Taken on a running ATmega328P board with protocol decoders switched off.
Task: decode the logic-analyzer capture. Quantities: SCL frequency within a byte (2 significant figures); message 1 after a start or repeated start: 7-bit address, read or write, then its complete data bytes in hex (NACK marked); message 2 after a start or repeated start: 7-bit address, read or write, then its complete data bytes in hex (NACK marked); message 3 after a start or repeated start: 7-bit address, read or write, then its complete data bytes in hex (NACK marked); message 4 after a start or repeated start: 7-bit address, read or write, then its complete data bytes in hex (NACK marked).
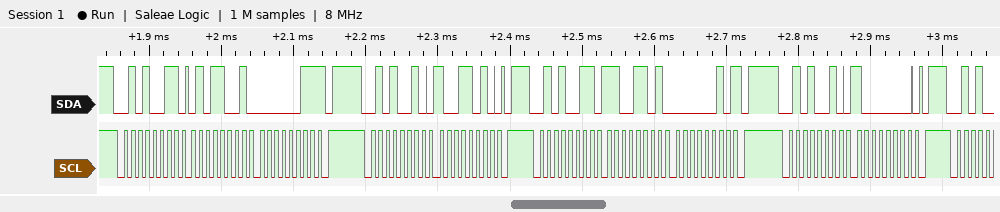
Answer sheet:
100 kHz
0x29 read: 59 03 NACK
0x29 write: 9A
0x29 read: CD 02 NACK
0x29 write: 80
